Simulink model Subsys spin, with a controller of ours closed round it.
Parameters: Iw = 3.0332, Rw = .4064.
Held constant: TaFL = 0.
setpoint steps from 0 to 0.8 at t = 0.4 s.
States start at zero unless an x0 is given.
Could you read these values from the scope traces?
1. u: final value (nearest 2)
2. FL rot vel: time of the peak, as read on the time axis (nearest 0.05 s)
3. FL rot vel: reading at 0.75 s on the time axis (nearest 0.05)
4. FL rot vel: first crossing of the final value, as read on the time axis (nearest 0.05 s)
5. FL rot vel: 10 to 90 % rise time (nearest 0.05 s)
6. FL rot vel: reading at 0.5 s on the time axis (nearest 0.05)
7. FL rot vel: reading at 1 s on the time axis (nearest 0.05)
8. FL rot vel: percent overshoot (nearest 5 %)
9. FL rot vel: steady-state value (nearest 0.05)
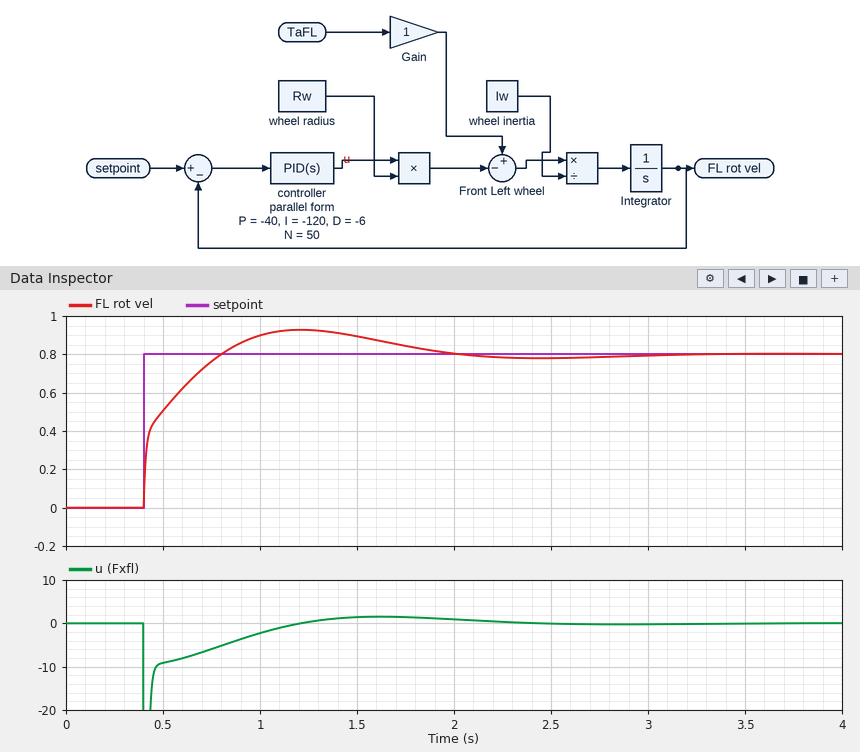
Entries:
0
1.20 s
0.75
0.80 s
0.30 s
0.50
0.90
15 %
0.80
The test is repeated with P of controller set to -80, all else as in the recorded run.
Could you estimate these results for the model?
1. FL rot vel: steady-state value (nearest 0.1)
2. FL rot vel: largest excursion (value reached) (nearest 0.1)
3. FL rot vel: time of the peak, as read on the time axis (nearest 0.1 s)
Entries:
0.8
0.9
1.1 s
